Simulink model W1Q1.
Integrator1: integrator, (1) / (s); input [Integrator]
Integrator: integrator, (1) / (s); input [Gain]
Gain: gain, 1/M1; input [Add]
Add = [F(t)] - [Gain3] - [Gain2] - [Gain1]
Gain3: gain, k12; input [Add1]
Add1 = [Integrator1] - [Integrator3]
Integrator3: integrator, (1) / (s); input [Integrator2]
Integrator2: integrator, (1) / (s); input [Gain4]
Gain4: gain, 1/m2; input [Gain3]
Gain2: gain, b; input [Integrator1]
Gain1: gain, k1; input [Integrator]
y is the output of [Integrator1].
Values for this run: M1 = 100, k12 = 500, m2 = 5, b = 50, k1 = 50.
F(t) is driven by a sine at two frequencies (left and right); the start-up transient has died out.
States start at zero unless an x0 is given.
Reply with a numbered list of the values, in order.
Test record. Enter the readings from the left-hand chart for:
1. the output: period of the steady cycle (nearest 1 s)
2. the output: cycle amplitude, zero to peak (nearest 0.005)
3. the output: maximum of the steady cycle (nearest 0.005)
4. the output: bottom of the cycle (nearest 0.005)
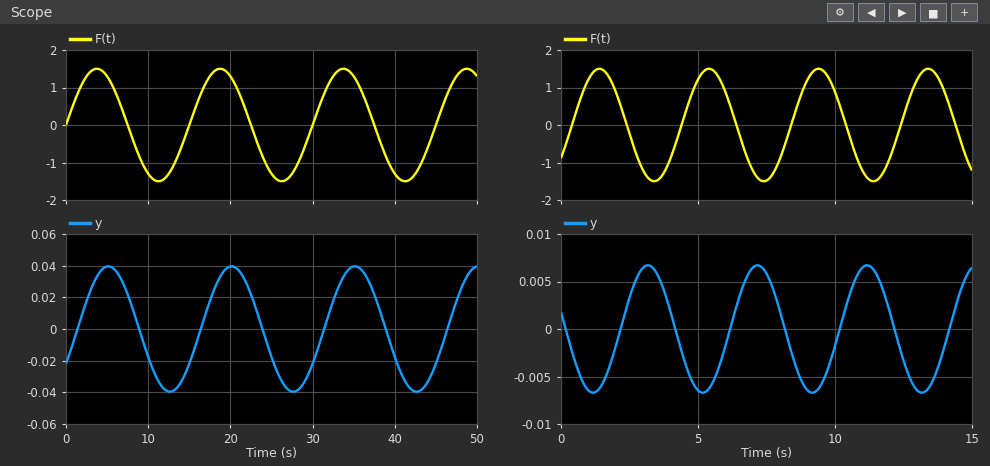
1. 15 s
2. 0.040
3. 0.040
4. -0.040
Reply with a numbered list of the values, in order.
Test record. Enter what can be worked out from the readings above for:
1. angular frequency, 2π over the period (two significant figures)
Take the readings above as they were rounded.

1. 0.42 rad/s
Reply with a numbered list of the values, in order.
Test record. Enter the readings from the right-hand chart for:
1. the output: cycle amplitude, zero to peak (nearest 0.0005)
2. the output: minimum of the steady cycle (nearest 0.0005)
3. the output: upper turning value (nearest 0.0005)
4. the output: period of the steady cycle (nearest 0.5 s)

1. 0.0065
2. -0.0065
3. 0.0065
4. 4.0 s
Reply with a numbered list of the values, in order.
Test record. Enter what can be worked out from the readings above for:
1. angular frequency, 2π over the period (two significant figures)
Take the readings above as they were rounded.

1. 1.6 rad/s
